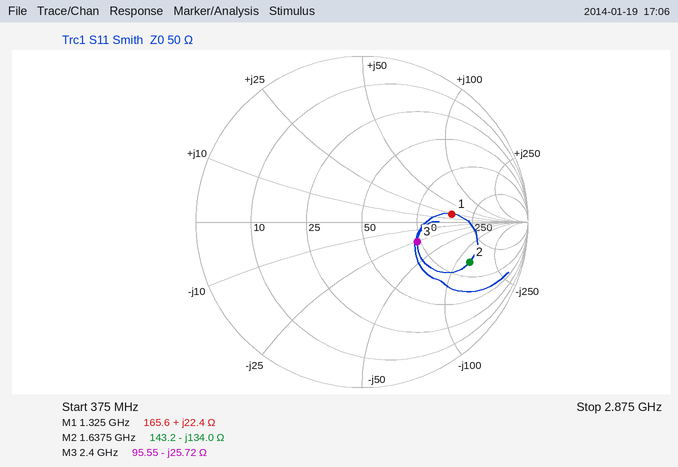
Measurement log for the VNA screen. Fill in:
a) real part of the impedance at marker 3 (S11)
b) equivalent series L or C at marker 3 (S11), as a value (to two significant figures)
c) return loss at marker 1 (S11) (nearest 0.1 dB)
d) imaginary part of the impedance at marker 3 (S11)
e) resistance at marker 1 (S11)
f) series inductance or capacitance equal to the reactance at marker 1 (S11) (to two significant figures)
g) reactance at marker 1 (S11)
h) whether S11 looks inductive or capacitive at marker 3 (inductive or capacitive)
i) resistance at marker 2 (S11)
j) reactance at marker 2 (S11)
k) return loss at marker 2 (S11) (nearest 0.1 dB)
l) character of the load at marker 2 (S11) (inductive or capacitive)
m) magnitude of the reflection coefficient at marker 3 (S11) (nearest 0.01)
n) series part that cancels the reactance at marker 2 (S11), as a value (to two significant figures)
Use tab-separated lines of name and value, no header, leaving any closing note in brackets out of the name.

real part of the impedance at marker 3	95.55 Ω
equivalent series L or C at marker 3 (S11), as a value	2.6 pF
return loss at marker 1 (S11)	5.3 dB
imaginary part of the impedance at marker 3	-25.72 Ω
resistance at marker 1	165.6 Ω
series inductance or capacitance equal to the reactance at marker 1 (S11)	2.7 nH
reactance at marker 1	+22.4 Ω
whether S11 looks inductive or capacitive at marker 3	capacitive
resistance at marker 2	143.2 Ω
reactance at marker 2	-134.0 Ω
return loss at marker 2 (S11)	3.2 dB
character of the load at marker 2 (S11)	capacitive
magnitude of the reflection coefficient at marker 3 (S11)	0.35
series part that cancels the reactance at marker 2 (S11), as a value	13 nH
